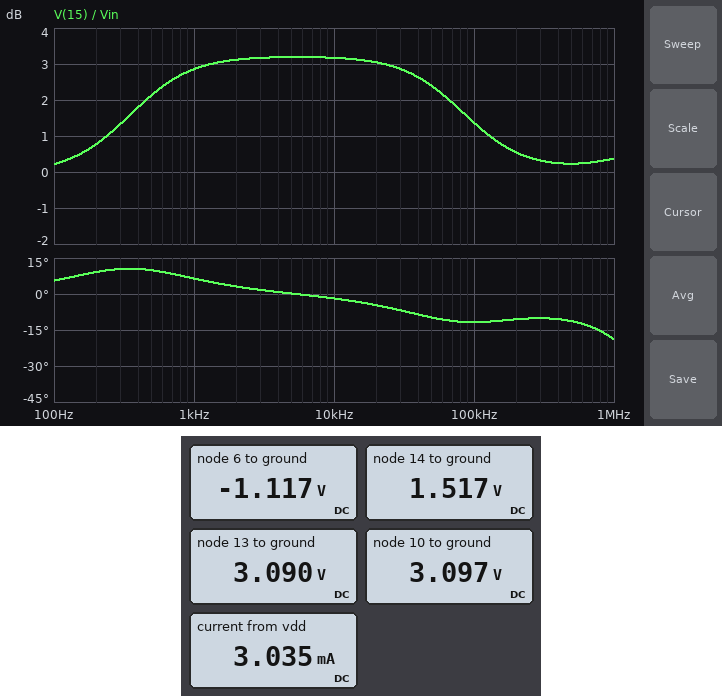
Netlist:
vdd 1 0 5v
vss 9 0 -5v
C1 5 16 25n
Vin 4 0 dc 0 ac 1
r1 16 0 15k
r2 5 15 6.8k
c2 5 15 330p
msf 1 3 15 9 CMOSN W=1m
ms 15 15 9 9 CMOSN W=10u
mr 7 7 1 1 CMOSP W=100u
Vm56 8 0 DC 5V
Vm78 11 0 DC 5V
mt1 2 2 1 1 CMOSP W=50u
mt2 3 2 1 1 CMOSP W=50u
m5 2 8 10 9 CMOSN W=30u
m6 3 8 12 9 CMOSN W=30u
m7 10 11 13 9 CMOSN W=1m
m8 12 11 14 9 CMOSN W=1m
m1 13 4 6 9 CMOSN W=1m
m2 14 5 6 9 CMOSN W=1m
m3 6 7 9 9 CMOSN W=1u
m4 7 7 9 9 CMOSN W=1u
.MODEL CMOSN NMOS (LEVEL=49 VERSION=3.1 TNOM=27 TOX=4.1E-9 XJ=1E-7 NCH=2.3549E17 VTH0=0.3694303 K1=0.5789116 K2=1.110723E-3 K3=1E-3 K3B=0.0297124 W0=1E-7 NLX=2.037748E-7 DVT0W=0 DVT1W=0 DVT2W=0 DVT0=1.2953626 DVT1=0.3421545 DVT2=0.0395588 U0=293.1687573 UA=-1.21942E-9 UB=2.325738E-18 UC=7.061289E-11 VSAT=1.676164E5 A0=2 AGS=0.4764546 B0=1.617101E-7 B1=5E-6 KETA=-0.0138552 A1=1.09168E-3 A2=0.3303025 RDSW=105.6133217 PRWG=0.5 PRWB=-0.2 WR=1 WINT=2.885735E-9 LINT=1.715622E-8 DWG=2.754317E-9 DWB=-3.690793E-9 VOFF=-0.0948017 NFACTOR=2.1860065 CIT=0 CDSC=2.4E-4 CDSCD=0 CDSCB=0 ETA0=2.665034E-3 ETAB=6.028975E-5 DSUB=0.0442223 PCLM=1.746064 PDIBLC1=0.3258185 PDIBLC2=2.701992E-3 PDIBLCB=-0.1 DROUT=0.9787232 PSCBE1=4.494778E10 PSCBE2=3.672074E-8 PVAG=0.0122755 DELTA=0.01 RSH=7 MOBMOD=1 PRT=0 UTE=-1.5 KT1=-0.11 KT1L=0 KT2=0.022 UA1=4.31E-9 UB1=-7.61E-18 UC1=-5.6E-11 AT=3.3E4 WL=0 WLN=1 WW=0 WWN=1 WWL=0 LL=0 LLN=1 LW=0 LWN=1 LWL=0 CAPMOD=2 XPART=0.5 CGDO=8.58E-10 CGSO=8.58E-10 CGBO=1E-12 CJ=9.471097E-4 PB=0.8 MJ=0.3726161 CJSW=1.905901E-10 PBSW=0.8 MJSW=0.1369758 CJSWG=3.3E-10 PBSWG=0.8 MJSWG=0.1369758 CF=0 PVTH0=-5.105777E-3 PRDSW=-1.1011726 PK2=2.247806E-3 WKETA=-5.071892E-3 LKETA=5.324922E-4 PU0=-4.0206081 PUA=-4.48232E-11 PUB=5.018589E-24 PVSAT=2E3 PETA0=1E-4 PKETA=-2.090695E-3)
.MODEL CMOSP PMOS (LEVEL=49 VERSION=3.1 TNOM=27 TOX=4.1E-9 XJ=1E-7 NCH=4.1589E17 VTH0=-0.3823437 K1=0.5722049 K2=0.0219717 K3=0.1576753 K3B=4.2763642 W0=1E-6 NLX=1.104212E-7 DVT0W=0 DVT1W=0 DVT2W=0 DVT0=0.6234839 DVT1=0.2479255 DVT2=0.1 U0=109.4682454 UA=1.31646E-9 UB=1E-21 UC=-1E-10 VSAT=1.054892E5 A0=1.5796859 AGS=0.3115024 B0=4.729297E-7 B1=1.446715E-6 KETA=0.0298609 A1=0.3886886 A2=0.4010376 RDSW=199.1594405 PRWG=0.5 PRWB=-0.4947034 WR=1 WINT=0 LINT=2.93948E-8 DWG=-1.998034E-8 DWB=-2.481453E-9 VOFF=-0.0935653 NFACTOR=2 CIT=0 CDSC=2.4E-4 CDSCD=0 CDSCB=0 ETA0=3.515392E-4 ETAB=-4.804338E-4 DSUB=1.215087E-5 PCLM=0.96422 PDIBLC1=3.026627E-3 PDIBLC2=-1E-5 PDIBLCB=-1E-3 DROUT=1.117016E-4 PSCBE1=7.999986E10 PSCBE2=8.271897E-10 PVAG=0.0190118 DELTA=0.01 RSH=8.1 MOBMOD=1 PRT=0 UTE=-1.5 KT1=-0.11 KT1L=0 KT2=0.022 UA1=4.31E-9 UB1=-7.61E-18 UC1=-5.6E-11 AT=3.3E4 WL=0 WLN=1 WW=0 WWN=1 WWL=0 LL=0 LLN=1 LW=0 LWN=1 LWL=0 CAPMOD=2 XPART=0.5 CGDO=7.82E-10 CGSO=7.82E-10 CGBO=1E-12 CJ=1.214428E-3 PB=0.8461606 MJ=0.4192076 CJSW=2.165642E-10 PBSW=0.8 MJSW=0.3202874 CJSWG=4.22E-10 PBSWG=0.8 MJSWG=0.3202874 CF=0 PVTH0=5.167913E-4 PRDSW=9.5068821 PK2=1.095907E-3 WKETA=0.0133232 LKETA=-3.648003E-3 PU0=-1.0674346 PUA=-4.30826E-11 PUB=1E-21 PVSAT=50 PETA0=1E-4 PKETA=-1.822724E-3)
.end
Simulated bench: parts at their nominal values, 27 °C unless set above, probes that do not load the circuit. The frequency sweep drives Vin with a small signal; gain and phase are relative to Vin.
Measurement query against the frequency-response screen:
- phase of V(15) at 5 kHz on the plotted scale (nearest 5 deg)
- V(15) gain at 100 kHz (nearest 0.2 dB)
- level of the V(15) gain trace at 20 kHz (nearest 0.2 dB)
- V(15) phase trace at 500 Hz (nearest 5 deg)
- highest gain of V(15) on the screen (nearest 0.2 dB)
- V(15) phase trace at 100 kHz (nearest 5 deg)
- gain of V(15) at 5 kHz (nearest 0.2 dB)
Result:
0 deg
1.4 dB
3.0 dB
10 deg
3.2 dB
-10 deg
3.2 dB
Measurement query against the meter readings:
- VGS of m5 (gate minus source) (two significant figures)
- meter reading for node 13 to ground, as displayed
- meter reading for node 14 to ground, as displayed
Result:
1.9 V
3.090 V
1.517 V
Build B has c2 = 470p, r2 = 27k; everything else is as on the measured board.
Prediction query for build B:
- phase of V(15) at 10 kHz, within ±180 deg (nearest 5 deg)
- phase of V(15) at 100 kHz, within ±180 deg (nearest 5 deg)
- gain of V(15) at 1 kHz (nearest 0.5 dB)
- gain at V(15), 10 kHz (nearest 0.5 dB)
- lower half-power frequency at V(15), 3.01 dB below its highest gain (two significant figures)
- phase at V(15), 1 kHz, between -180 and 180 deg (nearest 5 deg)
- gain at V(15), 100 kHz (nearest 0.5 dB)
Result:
-20 deg
-15 deg
8.5 dB
7.0 dB
340 Hz
10 deg
0.5 dB
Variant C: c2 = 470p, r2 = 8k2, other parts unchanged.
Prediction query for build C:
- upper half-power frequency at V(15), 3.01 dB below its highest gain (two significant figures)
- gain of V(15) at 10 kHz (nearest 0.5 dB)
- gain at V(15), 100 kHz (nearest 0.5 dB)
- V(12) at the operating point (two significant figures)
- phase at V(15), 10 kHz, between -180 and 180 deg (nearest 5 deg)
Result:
110 kHz
3.5 dB
1.0 dB
1.5 V
-5 deg
